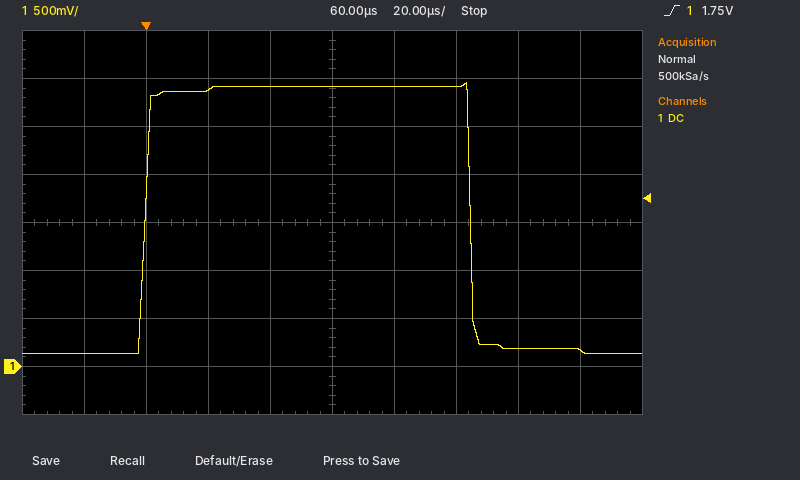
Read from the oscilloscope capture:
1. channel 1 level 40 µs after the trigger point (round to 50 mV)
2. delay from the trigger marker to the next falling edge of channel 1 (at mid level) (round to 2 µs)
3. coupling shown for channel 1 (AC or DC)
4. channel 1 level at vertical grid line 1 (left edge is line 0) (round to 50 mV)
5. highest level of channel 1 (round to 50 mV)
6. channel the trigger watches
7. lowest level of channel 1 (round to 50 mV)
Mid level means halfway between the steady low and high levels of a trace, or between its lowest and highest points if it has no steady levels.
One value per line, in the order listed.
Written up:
2.90 V
104 µs
DC
150 mV
2.95 V
channel 1
150 mV
